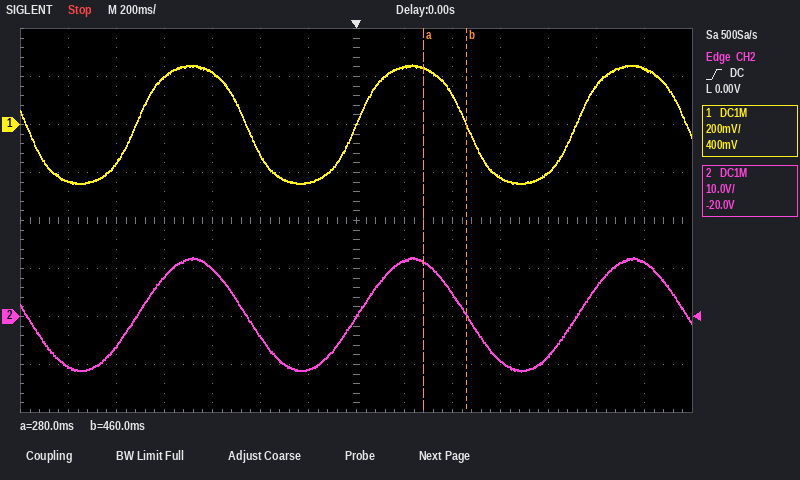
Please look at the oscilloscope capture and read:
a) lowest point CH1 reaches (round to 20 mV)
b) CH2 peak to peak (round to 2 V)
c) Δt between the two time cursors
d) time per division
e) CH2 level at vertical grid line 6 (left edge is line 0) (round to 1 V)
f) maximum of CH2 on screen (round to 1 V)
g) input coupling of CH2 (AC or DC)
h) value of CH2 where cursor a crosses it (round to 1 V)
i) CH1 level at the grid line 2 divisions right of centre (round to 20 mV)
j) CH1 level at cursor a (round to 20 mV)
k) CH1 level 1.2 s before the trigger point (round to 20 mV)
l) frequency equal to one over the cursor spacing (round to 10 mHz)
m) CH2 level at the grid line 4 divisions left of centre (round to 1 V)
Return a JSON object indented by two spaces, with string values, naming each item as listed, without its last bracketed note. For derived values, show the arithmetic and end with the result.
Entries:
{
  "lowest point CH1 reaches": "-240 mV",
  "CH2 peak to peak": "24 V",
  "Δt between the two time cursors": "460 ms − (280 ms) = 180 ms",
  "time per division": "200 ms",
  "CH2 level at vertical grid line 6 (left edge is line 0)": "-11 V",
  "maximum of CH2 on screen": "12 V",
  "input coupling of CH2": "DC",
  "value of CH2 where cursor a crosses it": "11 V",
  "CH1 level at the grid line 2 divisions right of centre": "120 mV",
  "CH1 level at cursor a": "240 mV",
  "CH1 level 1.2 s before the trigger point": "-240 mV",
  "frequency equal to one over the cursor spacing": "1 / 180 ms ≈ 5.56 Hz",
  "CH2 level at the grid line 4 divisions left of centre": "8 V"
}
